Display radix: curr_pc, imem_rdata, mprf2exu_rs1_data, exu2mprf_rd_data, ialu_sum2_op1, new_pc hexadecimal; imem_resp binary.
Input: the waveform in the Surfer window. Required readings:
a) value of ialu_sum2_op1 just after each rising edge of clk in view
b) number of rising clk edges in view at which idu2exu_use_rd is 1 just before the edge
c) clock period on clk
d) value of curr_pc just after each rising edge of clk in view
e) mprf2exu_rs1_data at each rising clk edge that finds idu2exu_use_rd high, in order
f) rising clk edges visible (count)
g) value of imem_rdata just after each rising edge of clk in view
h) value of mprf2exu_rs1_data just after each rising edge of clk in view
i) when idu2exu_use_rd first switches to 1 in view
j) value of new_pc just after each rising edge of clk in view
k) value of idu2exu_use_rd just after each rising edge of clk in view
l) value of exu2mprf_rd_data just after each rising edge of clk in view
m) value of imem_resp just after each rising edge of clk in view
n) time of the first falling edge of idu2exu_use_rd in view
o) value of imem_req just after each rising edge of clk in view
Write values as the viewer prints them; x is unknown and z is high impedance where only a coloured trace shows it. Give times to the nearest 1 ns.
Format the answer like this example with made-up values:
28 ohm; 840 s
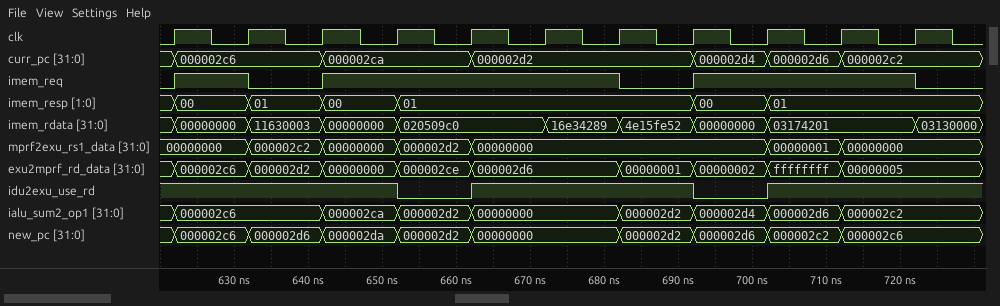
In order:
000002c6, 000002c6, 000002ca, 000002d2, 00000000, 00000000, 000002d2, 000002d4, 000002d6, 000002c2, 000002c2; 9; 10 ns; 000002c6, 000002c6, 000002ca, 000002ca, 000002d2, 000002d2, 000002d2, 000002d4, 000002d6, 000002c2, 000002c2; 00000000, 00000000, 000002c2, 00000000, 00000000, 00000000, 00000000, 00000001, 00000000; 11; 00000000, 11630003, 00000000, 020509c0, 020509c0, 16e34289, 4e15fe52, 00000000, 03174201, 03174201, 03130000; 00000000, 000002c2, 00000000, 000002d2, 00000000, 00000000, 00000000, 00000000, 00000001, 00000000, 00000000; 662 ns; 000002c6, 000002d6, 000002da, 000002d2, 00000000, 00000000, 000002d2, 000002d6, 000002c2, 000002c6, 000002c6; 1 1 1 0 1 1 1 0 1 1 1; 000002c6, 000002d2, 00000000, 000002ce, 000002d6, 000002d6, 00000001, 00000002, ffffffff, 00000005, 00000005; 00, 01, 00, 01, 01, 01, 01, 00, 01, 01, 01; 652 ns; 1 0 1 1 1 1 0 1 1 1 0
